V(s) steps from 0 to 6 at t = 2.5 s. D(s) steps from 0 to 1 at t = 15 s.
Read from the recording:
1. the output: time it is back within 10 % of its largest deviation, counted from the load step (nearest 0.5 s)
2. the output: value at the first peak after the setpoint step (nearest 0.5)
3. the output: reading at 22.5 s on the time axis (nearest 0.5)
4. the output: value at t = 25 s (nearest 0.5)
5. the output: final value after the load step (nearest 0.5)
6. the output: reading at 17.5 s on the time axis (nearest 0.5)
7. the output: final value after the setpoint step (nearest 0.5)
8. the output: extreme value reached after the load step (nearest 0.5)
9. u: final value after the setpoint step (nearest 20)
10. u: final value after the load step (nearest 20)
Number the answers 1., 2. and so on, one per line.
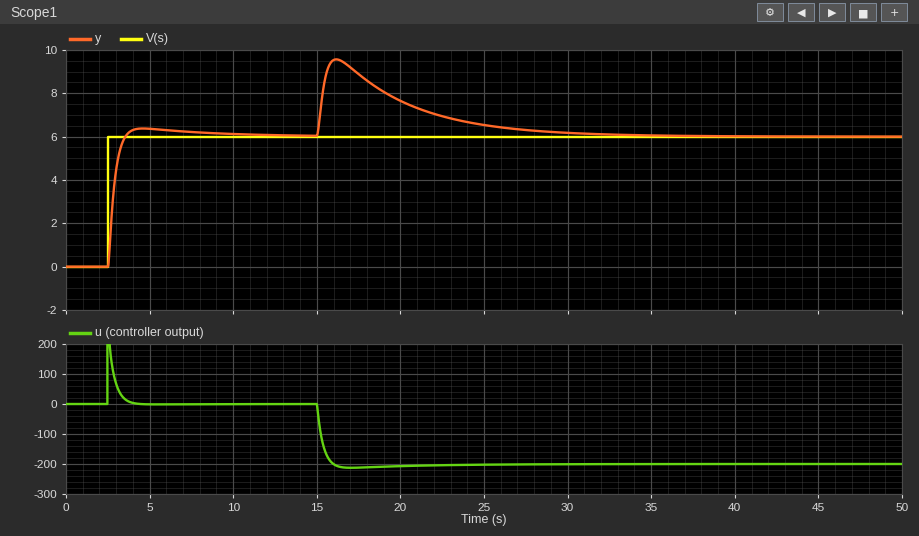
1. 12.0 s
2. 6.5
3. 7.0
4. 6.5
5. 6.0
6. 9.0
7. 6.0
8. 9.5
9. 0
10. -200
